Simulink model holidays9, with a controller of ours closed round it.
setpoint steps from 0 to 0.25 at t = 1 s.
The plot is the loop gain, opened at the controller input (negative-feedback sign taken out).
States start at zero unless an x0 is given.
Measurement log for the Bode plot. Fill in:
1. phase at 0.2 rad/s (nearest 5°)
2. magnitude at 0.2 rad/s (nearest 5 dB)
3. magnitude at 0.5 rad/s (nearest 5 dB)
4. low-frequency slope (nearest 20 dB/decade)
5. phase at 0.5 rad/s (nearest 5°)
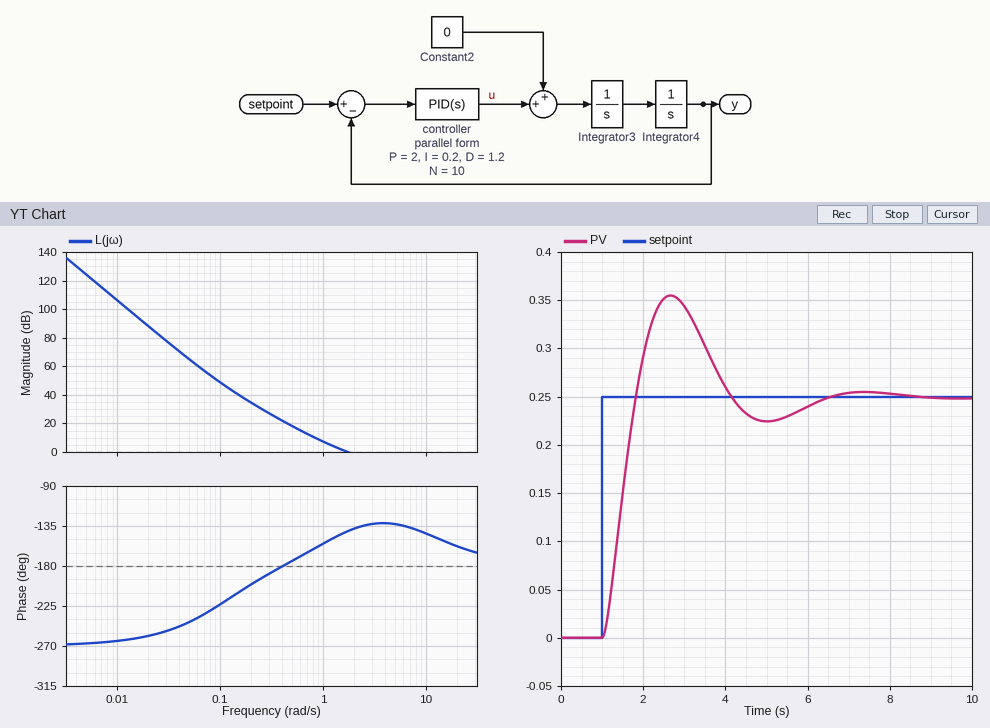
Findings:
-200°
35 dB
20 dB
-60 dB/decade
-175°
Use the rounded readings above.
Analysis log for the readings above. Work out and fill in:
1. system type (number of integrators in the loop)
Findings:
3
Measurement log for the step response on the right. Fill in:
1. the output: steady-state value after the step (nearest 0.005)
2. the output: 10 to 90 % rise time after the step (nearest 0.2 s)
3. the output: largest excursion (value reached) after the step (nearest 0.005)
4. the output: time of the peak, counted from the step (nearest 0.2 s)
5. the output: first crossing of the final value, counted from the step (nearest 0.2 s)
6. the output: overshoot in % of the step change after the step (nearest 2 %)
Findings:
0.250
0.6 s
0.355
1.6 s
0.8 s
42 %
